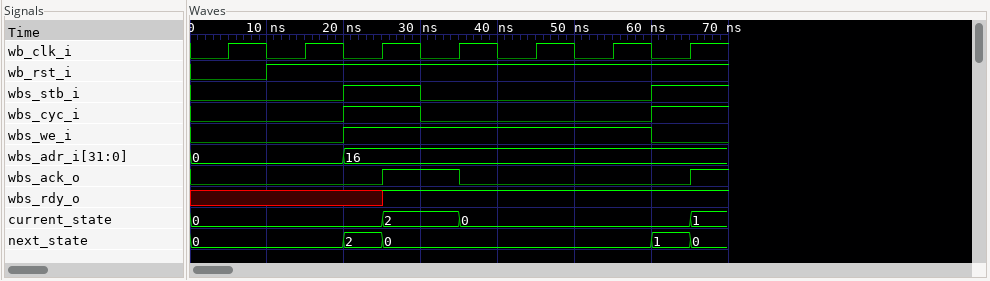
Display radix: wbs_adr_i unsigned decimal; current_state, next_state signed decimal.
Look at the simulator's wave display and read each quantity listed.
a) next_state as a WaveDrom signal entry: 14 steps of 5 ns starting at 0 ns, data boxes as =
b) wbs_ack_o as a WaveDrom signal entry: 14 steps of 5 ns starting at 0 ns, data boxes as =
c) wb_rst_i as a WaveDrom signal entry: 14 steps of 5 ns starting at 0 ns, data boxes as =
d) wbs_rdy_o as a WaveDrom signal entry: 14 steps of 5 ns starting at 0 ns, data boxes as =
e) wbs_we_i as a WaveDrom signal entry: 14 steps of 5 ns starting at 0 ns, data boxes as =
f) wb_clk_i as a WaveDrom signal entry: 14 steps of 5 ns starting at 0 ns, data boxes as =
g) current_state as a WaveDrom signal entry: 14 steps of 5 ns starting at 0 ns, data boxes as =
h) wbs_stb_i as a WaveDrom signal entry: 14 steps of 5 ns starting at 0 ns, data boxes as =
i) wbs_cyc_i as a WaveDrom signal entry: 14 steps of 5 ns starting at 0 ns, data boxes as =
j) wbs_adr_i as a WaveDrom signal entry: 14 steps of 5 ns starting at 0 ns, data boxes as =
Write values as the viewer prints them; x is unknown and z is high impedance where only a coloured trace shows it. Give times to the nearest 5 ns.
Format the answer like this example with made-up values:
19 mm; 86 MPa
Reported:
{name: 'next_state', wave: '=...==......==', data: '0 2 0 1 0'}; {name: 'wbs_ack_o', wave: '0....1.0.....1'}; {name: 'wb_rst_i', wave: '0.1...........'}; {name: 'wbs_rdy_o', wave: 'x....1........'}; {name: 'wbs_we_i', wave: '0...1.......0.'}; {name: 'wb_clk_i', wave: '01010101010101'}; {name: 'current_state', wave: '=....=.=.....=', data: '0 2 0 1'}; {name: 'wbs_stb_i', wave: '0...1.0.....1.'}; {name: 'wbs_cyc_i', wave: '0...1.0.....1.'}; {name: 'wbs_adr_i', wave: '=...=.........', data: '0 16'}
